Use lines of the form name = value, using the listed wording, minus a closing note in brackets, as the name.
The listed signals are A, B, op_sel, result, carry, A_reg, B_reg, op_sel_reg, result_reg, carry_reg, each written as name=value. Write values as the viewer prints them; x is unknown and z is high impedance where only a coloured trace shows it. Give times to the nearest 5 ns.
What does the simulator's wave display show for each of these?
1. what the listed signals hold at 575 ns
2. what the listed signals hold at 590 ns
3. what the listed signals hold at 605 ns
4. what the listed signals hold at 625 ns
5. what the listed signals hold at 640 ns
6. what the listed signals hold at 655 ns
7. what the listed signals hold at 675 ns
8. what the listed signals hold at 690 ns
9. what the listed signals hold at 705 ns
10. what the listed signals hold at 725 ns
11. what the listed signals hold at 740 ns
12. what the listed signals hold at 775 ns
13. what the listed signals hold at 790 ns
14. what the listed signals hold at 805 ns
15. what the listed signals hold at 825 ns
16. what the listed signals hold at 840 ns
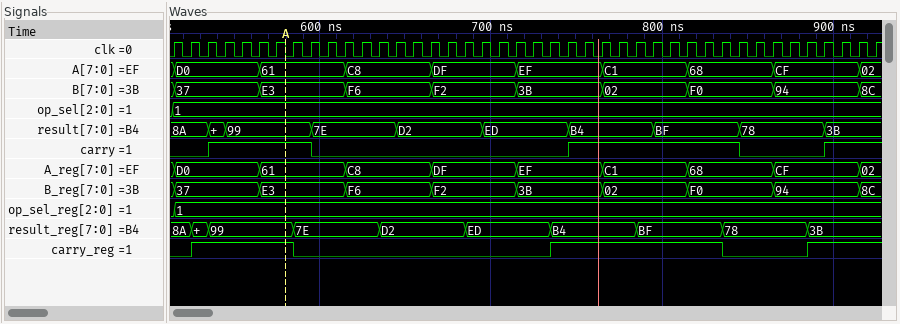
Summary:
what the listed signals hold at 575 ns = A=61, B=E3, op_sel=1, result=99, carry=1, A_reg=61, B_reg=E3, op_sel_reg=1, result_reg=99, carry_reg=1
what the listed signals hold at 590 ns = A=61, B=E3, op_sel=1, result=99, carry=1, A_reg=61, B_reg=E3, op_sel_reg=1, result_reg=7E, carry_reg=0
what the listed signals hold at 605 ns = A=61, B=E3, op_sel=1, result=7E, carry=0, A_reg=61, B_reg=E3, op_sel_reg=1, result_reg=7E, carry_reg=0
what the listed signals hold at 625 ns = A=C8, B=F6, op_sel=1, result=7E, carry=0, A_reg=C8, B_reg=F6, op_sel_reg=1, result_reg=7E, carry_reg=0
what the listed signals hold at 640 ns = A=C8, B=F6, op_sel=1, result=7E, carry=0, A_reg=C8, B_reg=F6, op_sel_reg=1, result_reg=D2, carry_reg=0
what the listed signals hold at 655 ns = A=C8, B=F6, op_sel=1, result=D2, carry=0, A_reg=C8, B_reg=F6, op_sel_reg=1, result_reg=D2, carry_reg=0
what the listed signals hold at 675 ns = A=DF, B=F2, op_sel=1, result=D2, carry=0, A_reg=DF, B_reg=F2, op_sel_reg=1, result_reg=D2, carry_reg=0
what the listed signals hold at 690 ns = A=DF, B=F2, op_sel=1, result=D2, carry=0, A_reg=DF, B_reg=F2, op_sel_reg=1, result_reg=ED, carry_reg=0
what the listed signals hold at 705 ns = A=DF, B=F2, op_sel=1, result=ED, carry=0, A_reg=DF, B_reg=F2, op_sel_reg=1, result_reg=ED, carry_reg=0
what the listed signals hold at 725 ns = A=EF, B=3B, op_sel=1, result=ED, carry=0, A_reg=EF, B_reg=3B, op_sel_reg=1, result_reg=ED, carry_reg=0
what the listed signals hold at 740 ns = A=EF, B=3B, op_sel=1, result=ED, carry=0, A_reg=EF, B_reg=3B, op_sel_reg=1, result_reg=B4, carry_reg=1
what the listed signals hold at 775 ns = A=C1, B=02, op_sel=1, result=B4, carry=1, A_reg=C1, B_reg=02, op_sel_reg=1, result_reg=B4, carry_reg=1
what the listed signals hold at 790 ns = A=C1, B=02, op_sel=1, result=B4, carry=1, A_reg=C1, B_reg=02, op_sel_reg=1, result_reg=BF, carry_reg=1
what the listed signals hold at 805 ns = A=C1, B=02, op_sel=1, result=BF, carry=1, A_reg=C1, B_reg=02, op_sel_reg=1, result_reg=BF, carry_reg=1
what the listed signals hold at 825 ns = A=68, B=F0, op_sel=1, result=BF, carry=1, A_reg=68, B_reg=F0, op_sel_reg=1, result_reg=BF, carry_reg=1
what the listed signals hold at 840 ns = A=68, B=F0, op_sel=1, result=BF, carry=1, A_reg=68, B_reg=F0, op_sel_reg=1, result_reg=78, carry_reg=0
